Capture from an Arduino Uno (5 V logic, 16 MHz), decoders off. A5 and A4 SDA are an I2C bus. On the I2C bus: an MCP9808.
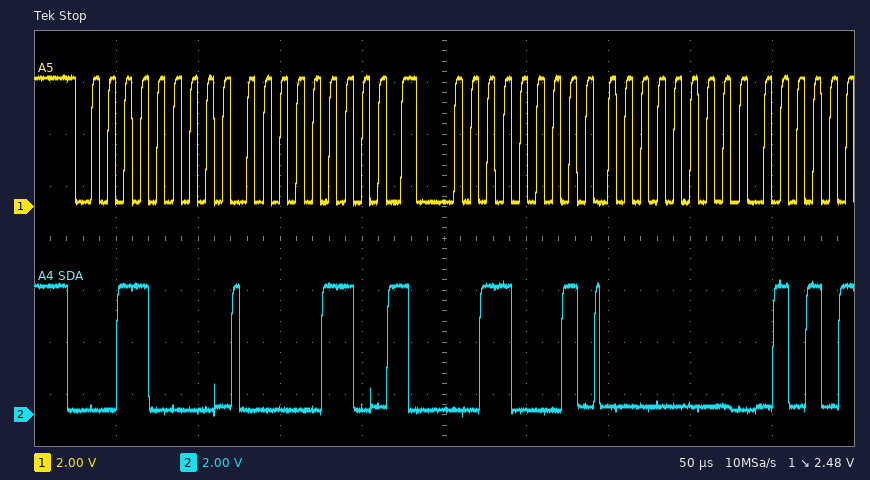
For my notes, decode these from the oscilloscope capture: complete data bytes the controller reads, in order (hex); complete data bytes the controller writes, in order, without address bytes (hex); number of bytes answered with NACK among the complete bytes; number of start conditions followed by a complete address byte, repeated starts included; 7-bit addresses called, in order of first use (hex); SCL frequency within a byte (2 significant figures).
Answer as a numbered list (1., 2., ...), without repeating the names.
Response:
1. 00
2. 06
3. 0
4. 2
5. 0x18
6. 100 kHz
